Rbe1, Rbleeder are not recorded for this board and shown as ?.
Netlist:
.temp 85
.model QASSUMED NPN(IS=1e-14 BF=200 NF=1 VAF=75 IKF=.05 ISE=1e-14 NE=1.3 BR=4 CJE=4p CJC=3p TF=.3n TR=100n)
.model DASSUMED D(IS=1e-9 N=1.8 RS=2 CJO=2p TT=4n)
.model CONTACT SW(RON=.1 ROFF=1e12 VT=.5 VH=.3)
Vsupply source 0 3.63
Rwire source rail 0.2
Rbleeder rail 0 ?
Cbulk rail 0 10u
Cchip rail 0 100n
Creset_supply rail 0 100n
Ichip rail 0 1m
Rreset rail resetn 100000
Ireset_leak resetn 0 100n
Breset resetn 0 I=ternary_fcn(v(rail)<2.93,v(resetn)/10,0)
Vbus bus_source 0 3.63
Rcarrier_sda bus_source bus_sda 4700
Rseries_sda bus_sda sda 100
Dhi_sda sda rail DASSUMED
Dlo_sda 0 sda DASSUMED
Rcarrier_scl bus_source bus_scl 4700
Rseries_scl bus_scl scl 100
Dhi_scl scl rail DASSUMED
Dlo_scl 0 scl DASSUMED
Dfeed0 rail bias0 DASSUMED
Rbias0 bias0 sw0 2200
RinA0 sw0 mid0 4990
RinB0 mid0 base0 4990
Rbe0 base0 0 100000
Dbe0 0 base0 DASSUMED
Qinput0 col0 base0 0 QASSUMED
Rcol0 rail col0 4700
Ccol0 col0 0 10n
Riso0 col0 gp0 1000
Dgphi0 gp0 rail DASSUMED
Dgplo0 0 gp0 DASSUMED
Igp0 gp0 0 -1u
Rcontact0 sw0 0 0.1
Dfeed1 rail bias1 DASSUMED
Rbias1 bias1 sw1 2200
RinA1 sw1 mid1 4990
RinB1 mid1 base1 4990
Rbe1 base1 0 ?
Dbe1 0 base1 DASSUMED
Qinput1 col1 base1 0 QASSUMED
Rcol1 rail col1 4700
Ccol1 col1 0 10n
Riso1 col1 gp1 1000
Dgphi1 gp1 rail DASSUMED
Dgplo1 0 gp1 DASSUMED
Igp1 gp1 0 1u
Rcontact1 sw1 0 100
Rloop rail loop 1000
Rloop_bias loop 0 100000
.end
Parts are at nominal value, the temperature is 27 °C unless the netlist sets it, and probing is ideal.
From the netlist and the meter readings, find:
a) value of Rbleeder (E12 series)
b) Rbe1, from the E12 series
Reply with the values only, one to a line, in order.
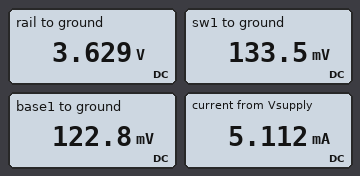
2.7 kΩ
120 kΩ
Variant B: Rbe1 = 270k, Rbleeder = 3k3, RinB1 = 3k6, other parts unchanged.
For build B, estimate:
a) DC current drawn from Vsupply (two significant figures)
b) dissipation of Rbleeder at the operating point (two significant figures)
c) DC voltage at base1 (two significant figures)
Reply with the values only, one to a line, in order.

4.9 mA
4.0 mW
130 mV
